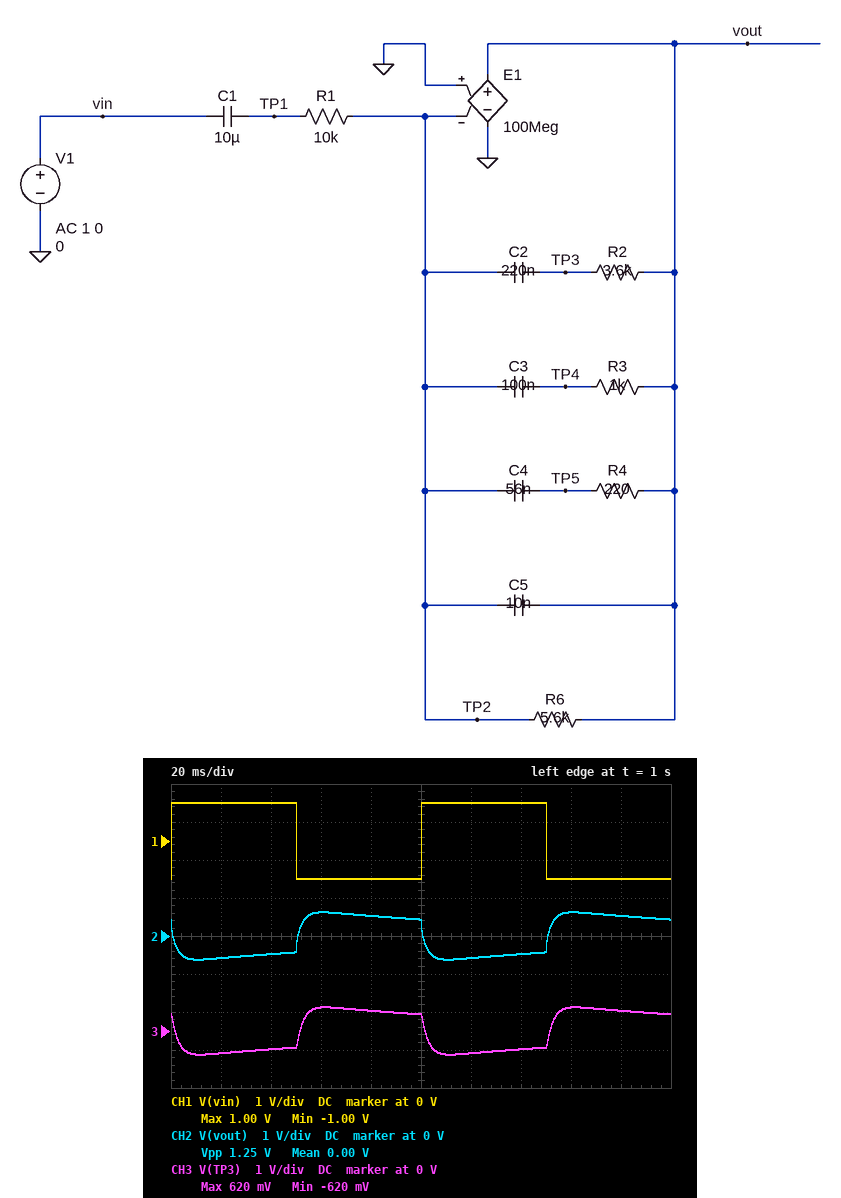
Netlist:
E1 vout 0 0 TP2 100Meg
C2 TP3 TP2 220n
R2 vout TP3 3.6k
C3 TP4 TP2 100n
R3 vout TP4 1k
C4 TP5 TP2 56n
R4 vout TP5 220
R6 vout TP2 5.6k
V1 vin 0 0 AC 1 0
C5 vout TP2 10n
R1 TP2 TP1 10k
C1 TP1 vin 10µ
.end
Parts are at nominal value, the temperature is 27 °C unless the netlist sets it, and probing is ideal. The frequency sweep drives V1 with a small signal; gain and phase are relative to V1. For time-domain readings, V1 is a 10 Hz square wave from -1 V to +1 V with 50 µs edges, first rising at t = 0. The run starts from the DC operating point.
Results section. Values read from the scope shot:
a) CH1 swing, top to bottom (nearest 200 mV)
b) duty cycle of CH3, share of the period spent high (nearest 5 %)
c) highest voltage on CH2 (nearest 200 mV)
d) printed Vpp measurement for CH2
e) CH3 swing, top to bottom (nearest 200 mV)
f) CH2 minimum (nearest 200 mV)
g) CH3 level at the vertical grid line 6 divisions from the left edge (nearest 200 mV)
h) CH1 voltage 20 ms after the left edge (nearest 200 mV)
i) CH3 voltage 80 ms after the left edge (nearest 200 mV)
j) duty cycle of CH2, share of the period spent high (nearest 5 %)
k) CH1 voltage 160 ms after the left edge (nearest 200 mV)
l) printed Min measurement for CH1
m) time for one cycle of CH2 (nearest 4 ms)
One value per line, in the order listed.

2.0 V
50 %
600 mV
1.25 V
1.2 V
-600 mV
-600 mV
1.0 V
600 mV
50 %
-1.0 V
-1.00 V
100 ms
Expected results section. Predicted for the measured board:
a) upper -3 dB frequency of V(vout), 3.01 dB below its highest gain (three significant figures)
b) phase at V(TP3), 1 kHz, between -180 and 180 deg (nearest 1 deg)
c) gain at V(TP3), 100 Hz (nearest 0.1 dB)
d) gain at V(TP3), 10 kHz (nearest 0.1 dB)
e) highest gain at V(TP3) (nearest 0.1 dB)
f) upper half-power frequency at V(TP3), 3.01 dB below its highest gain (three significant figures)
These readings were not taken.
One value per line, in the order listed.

67.3 Hz
51 deg
-11.1 dB
-66.7 dB
-5.3 dB
61.3 Hz
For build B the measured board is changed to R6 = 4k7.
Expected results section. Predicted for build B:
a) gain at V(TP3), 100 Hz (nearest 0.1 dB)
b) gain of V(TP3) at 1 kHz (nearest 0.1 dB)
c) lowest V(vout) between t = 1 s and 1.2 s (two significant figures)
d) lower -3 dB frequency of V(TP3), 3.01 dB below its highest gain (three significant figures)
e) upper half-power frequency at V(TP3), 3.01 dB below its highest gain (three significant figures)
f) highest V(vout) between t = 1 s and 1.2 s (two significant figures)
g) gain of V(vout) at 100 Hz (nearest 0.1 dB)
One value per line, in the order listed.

-11.8 dB
-35.8 dB
-530 mV
1.52 Hz
69.4 Hz
530 mV
-10.8 dB
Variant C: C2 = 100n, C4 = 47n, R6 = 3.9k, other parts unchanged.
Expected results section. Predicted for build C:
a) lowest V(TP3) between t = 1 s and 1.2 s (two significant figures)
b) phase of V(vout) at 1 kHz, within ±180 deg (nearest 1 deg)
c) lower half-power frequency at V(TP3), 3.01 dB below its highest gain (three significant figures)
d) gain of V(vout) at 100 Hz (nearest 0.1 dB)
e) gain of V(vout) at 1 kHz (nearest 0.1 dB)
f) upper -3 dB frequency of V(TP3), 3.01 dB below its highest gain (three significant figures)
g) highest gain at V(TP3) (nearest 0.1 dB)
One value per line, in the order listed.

-460 mV
131 deg
1.55 Hz
-10.0 dB
-21.6 dB
131 Hz
-8.3 dB
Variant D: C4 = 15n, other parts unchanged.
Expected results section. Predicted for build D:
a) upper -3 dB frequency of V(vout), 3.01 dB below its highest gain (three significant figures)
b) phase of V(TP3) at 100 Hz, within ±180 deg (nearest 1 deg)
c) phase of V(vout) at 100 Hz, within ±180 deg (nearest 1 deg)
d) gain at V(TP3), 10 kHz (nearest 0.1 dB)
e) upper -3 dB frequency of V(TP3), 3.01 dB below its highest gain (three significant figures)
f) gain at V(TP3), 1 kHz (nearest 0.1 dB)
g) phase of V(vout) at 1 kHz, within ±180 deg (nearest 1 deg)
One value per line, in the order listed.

73.0 Hz
116 deg
142 deg
-61.3 dB
65.5 Hz
-34.0 dB
138 deg
